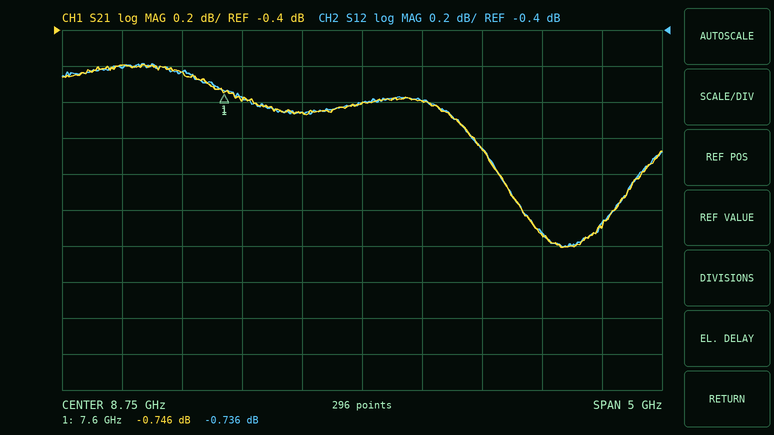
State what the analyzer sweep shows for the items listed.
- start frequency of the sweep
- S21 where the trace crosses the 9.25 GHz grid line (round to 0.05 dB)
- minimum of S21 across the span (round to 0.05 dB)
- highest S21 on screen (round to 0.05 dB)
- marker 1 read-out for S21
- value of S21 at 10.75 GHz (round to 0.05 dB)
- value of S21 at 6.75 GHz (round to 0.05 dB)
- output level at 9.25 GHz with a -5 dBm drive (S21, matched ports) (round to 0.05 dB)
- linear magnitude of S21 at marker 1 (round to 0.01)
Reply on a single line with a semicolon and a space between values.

6.25 GHz; -0.80 dB; -1.60 dB; -0.60 dB; -0.746 dB; -1.50 dB; -0.60 dB; -5.80 dBm; 0.92
